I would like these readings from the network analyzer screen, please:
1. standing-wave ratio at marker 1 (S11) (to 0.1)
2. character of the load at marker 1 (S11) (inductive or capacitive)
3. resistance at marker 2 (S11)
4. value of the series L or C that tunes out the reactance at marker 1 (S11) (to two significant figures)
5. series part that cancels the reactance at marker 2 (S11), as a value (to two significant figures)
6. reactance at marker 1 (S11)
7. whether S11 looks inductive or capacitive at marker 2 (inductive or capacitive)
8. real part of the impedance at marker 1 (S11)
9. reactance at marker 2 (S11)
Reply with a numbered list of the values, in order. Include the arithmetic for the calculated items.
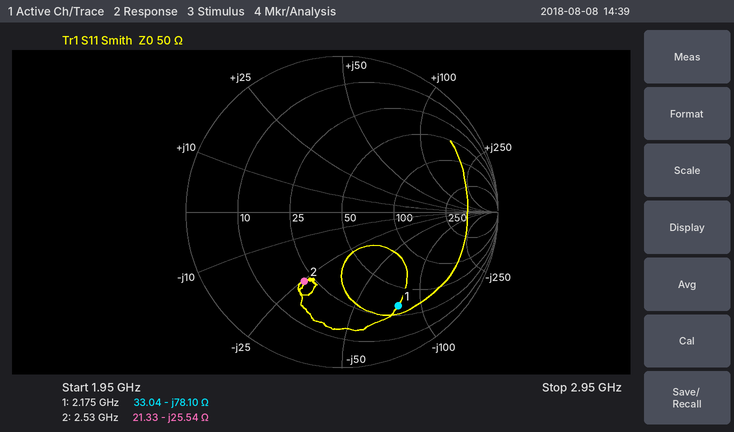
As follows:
1. 5.7
2. capacitive
3. 21.33 Ω
4. L = 78.1 Ω/(2π × 2.175 GHz) ≈ 5.7 nH
5. L = 25.54 Ω/(2π × 2.53 GHz) ≈ 1.6 nH
6. -78.10 Ω
7. capacitive
8. 33.04 Ω
9. -25.54 Ω
